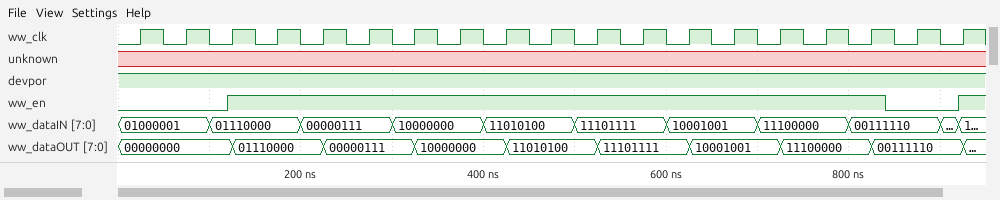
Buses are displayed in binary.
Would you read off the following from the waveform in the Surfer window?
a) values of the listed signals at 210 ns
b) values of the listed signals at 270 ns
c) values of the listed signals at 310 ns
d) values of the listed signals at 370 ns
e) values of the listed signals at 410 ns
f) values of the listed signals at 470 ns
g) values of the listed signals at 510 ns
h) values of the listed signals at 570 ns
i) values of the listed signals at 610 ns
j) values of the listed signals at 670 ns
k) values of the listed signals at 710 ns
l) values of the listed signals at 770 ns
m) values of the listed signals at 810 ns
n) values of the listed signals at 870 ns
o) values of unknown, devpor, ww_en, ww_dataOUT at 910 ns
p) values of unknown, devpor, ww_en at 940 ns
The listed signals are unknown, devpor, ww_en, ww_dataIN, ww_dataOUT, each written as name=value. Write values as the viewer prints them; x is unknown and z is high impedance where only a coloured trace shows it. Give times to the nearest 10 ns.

unknown=x, devpor=1, ww_en=1, ww_dataIN=00000111, ww_dataOUT=01110000
unknown=x, devpor=1, ww_en=1, ww_dataIN=00000111, ww_dataOUT=00000111
unknown=x, devpor=1, ww_en=1, ww_dataIN=10000000, ww_dataOUT=00000111
unknown=x, devpor=1, ww_en=1, ww_dataIN=10000000, ww_dataOUT=10000000
unknown=x, devpor=1, ww_en=1, ww_dataIN=11010100, ww_dataOUT=10000000
unknown=x, devpor=1, ww_en=1, ww_dataIN=11010100, ww_dataOUT=11010100
unknown=x, devpor=1, ww_en=1, ww_dataIN=11101111, ww_dataOUT=11010100
unknown=x, devpor=1, ww_en=1, ww_dataIN=11101111, ww_dataOUT=11101111
unknown=x, devpor=1, ww_en=1, ww_dataIN=10001001, ww_dataOUT=11101111
unknown=x, devpor=1, ww_en=1, ww_dataIN=10001001, ww_dataOUT=10001001
unknown=x, devpor=1, ww_en=1, ww_dataIN=11100000, ww_dataOUT=10001001
unknown=x, devpor=1, ww_en=1, ww_dataIN=11100000, ww_dataOUT=11100000
unknown=x, devpor=1, ww_en=1, ww_dataIN=00111110, ww_dataOUT=11100000
unknown=x, devpor=1, ww_en=0, ww_dataIN=00111110, ww_dataOUT=00111110
unknown=x, devpor=1, ww_en=0, ww_dataOUT=00111110
unknown=x, devpor=1, ww_en=1
